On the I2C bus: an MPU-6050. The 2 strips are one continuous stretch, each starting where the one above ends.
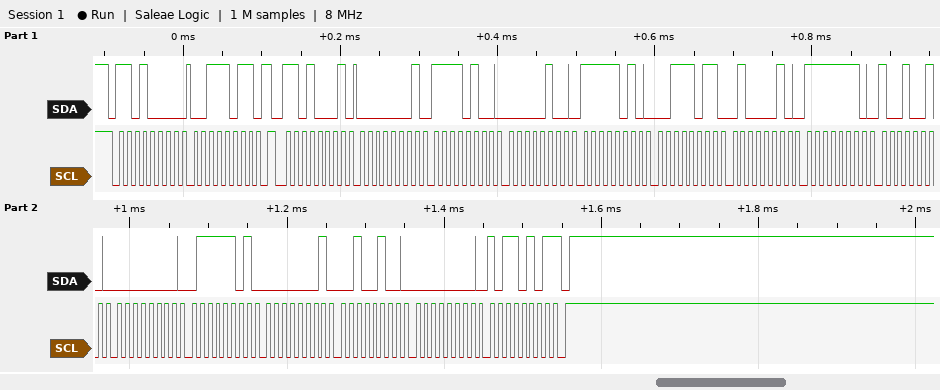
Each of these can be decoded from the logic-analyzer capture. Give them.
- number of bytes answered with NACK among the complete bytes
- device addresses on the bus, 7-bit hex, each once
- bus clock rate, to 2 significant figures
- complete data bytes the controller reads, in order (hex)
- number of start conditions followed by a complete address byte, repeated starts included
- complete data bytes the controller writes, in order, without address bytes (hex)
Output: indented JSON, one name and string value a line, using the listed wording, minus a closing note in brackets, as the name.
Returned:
{
  "number of bytes answered with NACK among the complete bytes": "1",
  "device addresses on the bus, 7-bit hex, each once": "0x68",
  "bus clock rate, to 2 significant figures": "100 kHz",
  "complete data bytes the controller reads, in order": "01 F4 04 FA 3B 42 FE 92 00 7D 01 24 00 B5",
  "number of start conditions followed by a complete address byte, repeated starts included": "2",
  "complete data bytes the controller writes, in order, without address bytes": "3B"
}
